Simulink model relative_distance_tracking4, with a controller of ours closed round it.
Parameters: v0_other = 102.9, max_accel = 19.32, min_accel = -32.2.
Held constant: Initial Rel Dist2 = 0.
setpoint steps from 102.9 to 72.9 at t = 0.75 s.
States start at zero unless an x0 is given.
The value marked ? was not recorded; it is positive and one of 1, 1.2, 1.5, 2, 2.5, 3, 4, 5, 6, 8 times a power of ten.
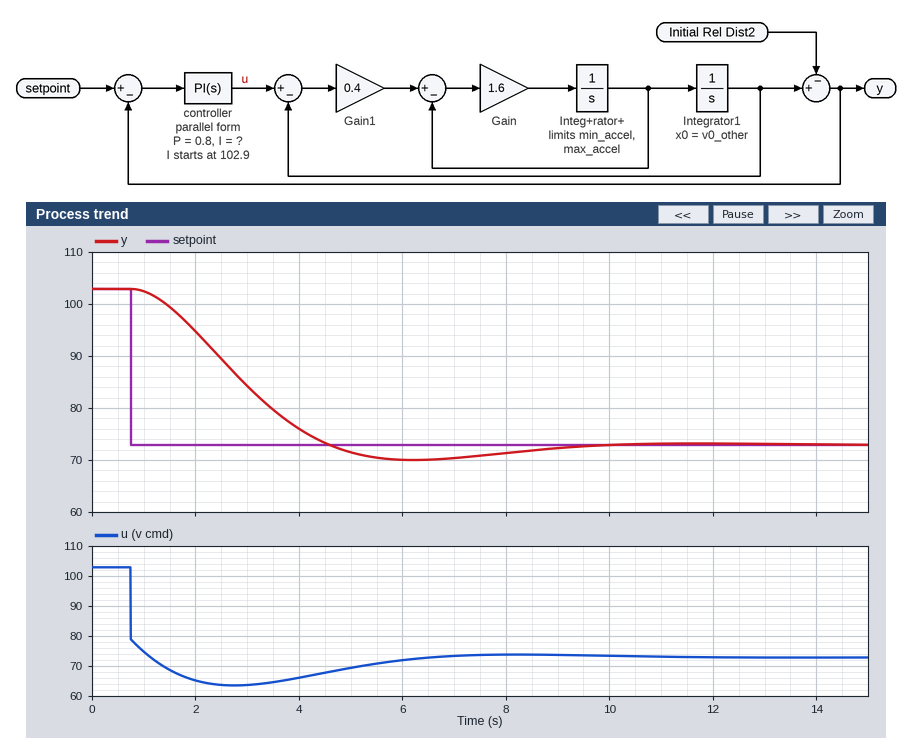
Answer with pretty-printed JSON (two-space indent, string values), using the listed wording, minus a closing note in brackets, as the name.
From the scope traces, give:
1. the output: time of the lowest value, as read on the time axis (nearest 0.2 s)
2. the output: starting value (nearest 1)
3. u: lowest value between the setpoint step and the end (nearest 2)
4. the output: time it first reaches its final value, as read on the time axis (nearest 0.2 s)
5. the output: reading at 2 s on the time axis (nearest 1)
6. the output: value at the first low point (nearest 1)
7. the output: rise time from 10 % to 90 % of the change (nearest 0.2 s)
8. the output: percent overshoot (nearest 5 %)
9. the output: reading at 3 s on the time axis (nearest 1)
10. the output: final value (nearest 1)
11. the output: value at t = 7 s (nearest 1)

{
  "the output: time of the lowest value, as read on the time axis": "6.2 s",
  "the output: starting value": "103",
  "u: lowest value between the setpoint step and the end": "64",
  "the output: time it first reaches its final value, as read on the time axis": "4.6 s",
  "the output: reading at 2 s on the time axis": "95",
  "the output: value at the first low point": "70",
  "the output: rise time from 10 % to 90 % of the change": "2.6 s",
  "the output: percent overshoot": "10 %",
  "the output: reading at 3 s on the time axis": "84",
  "the output: final value": "73",
  "the output: value at t = 7 s": "70"
}
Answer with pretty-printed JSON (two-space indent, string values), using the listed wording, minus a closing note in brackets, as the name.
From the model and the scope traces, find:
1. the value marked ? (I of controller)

{
  "the value marked ?": "0.6"
}
